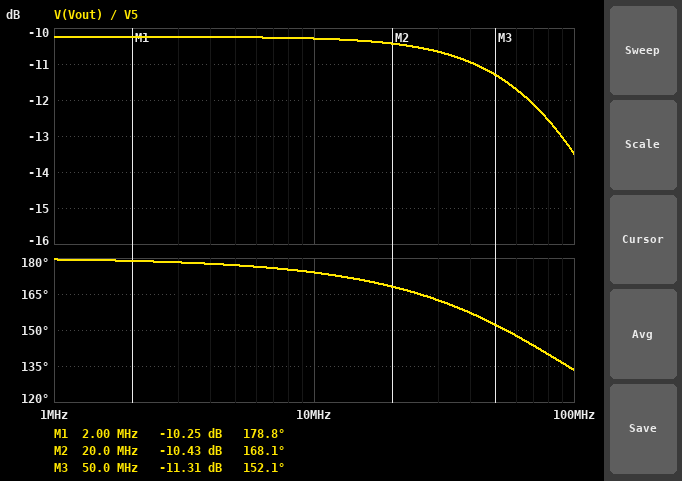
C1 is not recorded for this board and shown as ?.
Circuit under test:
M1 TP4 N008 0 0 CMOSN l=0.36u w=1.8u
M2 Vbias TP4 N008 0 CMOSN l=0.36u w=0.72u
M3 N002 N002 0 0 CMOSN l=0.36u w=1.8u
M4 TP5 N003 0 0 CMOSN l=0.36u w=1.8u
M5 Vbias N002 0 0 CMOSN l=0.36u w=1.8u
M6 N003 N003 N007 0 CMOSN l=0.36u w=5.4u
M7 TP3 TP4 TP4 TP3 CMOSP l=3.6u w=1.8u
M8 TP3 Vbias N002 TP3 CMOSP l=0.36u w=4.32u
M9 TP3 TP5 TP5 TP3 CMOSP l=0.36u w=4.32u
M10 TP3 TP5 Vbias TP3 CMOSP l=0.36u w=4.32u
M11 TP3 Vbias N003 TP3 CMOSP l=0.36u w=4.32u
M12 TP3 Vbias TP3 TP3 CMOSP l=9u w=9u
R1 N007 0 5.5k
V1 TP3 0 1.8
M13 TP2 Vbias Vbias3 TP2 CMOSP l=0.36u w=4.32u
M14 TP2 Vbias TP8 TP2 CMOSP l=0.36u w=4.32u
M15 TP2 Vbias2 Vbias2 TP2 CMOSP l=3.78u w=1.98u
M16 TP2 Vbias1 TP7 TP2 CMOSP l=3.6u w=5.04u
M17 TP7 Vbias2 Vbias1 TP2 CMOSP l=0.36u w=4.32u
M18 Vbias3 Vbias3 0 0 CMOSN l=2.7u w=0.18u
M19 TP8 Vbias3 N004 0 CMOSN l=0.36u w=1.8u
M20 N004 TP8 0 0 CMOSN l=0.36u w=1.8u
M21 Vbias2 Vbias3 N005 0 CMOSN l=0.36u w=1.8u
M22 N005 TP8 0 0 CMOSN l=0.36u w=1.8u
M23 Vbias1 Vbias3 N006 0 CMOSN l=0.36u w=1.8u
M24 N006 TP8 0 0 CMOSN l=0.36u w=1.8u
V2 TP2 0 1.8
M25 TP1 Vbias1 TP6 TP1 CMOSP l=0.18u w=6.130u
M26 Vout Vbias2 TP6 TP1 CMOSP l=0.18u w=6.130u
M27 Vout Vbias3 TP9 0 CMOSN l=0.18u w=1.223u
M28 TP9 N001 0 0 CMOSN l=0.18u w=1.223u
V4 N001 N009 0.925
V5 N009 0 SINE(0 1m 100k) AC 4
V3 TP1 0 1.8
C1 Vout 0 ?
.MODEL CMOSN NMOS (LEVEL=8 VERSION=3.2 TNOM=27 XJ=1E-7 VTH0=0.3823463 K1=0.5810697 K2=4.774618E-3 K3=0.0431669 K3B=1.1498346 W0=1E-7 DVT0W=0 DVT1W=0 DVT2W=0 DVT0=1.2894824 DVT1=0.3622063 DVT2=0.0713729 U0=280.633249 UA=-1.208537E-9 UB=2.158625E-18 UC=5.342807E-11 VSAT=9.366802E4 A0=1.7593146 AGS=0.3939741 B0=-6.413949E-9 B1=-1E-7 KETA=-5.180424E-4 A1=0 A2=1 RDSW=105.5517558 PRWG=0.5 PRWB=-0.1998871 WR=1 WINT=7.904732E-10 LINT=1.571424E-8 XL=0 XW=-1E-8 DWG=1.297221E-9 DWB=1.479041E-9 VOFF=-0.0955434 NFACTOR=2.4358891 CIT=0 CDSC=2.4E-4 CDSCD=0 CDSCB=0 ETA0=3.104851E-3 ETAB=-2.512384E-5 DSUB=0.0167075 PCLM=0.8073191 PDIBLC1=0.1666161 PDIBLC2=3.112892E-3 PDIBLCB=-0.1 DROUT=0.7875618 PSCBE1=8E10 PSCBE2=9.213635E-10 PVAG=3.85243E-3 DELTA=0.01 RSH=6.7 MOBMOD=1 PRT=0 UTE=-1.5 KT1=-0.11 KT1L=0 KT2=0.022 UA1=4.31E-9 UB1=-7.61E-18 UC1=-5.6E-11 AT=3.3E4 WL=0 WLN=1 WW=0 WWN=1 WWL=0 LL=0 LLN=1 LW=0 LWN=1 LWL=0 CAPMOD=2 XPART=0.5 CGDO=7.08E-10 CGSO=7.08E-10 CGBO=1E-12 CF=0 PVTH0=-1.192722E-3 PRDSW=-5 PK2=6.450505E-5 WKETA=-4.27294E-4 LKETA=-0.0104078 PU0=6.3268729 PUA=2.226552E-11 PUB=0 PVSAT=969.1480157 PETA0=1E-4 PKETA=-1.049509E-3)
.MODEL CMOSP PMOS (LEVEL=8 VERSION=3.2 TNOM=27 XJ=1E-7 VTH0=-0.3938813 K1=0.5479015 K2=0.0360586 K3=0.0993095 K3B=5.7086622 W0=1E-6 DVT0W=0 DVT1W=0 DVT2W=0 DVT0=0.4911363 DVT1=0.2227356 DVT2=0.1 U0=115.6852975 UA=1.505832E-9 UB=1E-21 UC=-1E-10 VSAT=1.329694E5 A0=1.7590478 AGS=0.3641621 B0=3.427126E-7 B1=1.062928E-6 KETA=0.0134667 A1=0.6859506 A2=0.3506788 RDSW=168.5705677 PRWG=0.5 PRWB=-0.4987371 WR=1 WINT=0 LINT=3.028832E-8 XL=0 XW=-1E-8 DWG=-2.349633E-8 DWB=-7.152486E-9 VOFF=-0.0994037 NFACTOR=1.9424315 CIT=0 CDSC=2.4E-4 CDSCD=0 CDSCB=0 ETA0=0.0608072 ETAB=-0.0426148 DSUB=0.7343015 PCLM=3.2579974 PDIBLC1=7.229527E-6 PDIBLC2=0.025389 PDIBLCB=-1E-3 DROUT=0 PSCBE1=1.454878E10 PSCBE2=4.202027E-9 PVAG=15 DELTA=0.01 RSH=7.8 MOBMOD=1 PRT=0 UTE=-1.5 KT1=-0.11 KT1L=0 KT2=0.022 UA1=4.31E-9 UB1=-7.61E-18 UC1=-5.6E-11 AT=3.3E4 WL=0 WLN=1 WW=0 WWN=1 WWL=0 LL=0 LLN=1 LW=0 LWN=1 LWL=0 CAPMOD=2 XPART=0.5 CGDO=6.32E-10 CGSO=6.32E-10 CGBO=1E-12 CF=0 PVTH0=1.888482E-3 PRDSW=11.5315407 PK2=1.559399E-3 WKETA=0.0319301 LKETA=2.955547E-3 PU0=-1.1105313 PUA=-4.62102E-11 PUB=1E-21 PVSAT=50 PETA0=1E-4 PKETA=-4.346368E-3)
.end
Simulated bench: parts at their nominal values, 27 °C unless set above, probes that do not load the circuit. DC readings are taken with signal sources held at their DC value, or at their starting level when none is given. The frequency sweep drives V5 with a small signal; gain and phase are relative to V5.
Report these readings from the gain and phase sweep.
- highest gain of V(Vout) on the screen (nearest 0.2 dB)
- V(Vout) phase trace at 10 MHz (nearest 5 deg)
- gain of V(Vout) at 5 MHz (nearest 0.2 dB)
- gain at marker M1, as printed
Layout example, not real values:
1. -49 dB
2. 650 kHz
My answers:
1. -10.2 dB
2. 175 deg
3. -10.2 dB
4. -10.25 dB
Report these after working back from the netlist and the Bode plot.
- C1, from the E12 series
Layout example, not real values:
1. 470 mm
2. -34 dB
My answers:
1. 3.3 pF
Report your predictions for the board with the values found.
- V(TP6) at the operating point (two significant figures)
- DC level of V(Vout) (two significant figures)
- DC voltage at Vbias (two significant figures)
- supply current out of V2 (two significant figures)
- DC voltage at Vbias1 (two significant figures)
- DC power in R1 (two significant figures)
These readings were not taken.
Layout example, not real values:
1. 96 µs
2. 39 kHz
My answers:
1. 1.8 V
2. 1.6 V
3. 1.8 V
4. 1.3 mA
5. 1.7 V
6. 140 µW
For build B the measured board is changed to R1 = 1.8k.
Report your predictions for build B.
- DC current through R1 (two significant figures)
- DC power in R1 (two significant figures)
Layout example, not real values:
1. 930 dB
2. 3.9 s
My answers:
1. 400 µA
2. 290 µW
